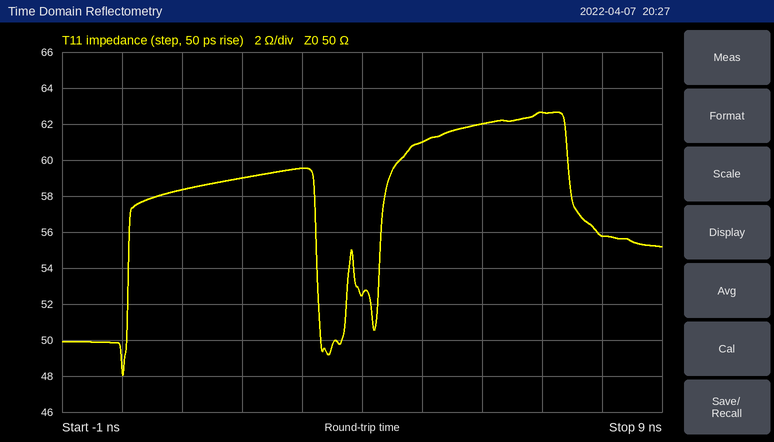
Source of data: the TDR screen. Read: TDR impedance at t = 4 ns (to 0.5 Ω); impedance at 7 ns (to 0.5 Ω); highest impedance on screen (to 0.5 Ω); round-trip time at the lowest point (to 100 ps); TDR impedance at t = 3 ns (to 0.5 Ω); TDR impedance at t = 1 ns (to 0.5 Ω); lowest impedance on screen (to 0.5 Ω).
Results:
52.5 Ω
62.5 Ω
62.5 Ω
0.0 ns
59.5 Ω
58.5 Ω
48.0 Ω
